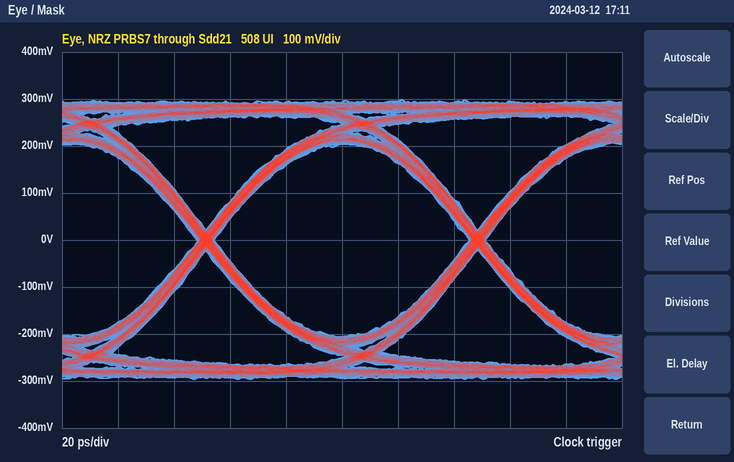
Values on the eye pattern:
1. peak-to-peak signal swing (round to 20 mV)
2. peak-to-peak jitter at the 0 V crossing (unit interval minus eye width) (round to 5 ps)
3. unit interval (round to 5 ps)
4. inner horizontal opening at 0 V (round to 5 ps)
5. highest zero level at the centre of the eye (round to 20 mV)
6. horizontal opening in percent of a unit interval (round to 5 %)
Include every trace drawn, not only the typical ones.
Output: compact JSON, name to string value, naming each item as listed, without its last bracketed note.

{"peak-to-peak signal swing": "600 mV", "peak-to-peak jitter at the 0 V crossing (unit interval minus eye width)": "5 ps", "unit interval": "95 ps", "inner horizontal opening at 0 V": "90 ps", "highest zero level at the centre of the eye": "-200 mV", "horizontal opening in percent of a unit interval": "95 %"}
